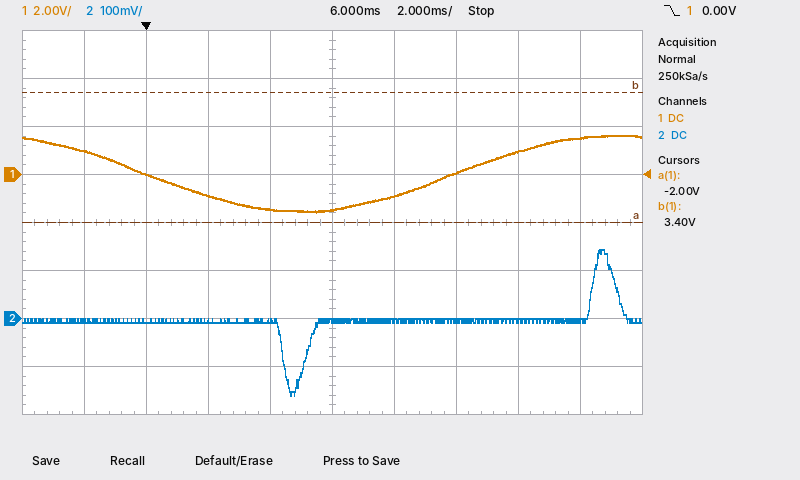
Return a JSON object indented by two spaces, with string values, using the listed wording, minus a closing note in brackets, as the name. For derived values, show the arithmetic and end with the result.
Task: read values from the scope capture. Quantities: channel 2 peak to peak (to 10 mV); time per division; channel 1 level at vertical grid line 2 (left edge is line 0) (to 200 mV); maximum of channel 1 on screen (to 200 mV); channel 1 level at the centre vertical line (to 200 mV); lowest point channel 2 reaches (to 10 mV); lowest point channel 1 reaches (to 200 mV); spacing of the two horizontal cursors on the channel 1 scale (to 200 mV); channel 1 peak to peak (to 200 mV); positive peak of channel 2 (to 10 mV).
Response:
{
  "channel 2 peak to peak": "140 mV − (-160 mV) = 300 mV",
  "time per division": "2 ms",
  "channel 1 level at vertical grid line 2 (left edge is line 0)": "0.0 V",
  "maximum of channel 1 on screen": "1.6 V",
  "channel 1 level at the centre vertical line": "-1.4 V",
  "lowest point channel 2 reaches": "-160 mV",
  "lowest point channel 1 reaches": "-1.6 V",
  "spacing of the two horizontal cursors on the channel 1 scale": "5.4 V",
  "channel 1 peak to peak": "1.6 V − (-1.6 V) = 3.2 V",
  "positive peak of channel 2": "140 mV"
}
